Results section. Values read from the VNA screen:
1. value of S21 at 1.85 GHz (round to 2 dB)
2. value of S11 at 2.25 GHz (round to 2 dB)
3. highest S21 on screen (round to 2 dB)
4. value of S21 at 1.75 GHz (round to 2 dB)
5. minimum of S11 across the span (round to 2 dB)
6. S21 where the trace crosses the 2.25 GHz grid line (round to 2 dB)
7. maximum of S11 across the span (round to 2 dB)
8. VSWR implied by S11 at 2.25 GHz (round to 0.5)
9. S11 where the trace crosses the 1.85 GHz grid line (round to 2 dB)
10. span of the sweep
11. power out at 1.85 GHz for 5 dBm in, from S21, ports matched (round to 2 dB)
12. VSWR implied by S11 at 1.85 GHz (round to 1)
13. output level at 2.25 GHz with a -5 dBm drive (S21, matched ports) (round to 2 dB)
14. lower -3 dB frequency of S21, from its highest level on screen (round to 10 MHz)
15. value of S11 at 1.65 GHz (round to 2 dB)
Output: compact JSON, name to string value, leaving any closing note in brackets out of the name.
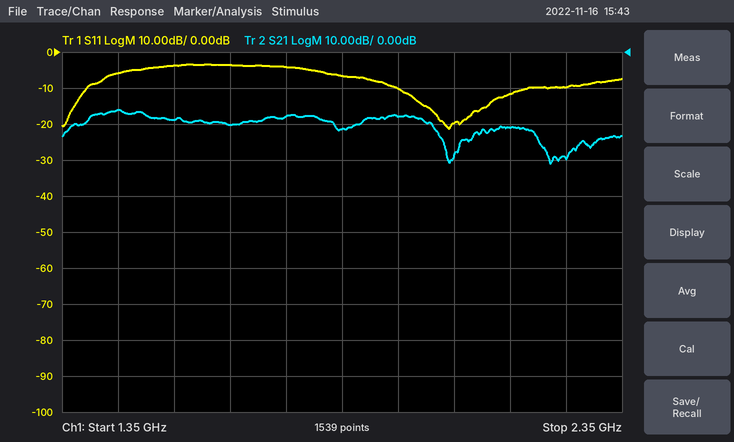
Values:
{"value of S21 at 1.85 GHz": "-22 dB", "value of S11 at 2.25 GHz": "-10 dB", "highest S21 on screen": "-16 dB", "value of S21 at 1.75 GHz": "-18 dB", "minimum of S11 across the span": "-22 dB", "S21 where the trace crosses the 2.25 GHz grid line": "-30 dB", "maximum of S11 across the span": "-4 dB", "VSWR implied by S11 at 2.25 GHz": "2.0", "S11 where the trace crosses the 1.85 GHz grid line": "-6 dB", "span of the sweep": "1 GHz", "power out at 1.85 GHz for 5 dBm in, from S21, ports matched": "-16 dBm", "VSWR implied by S11 at 1.85 GHz": "3", "output level at 2.25 GHz with a -5 dBm drive (S21, matched ports)": "-34 dBm", "lower -3 dB frequency of S21, from its highest level on screen": "1.40 GHz", "value of S11 at 1.65 GHz": "-4 dB"}
